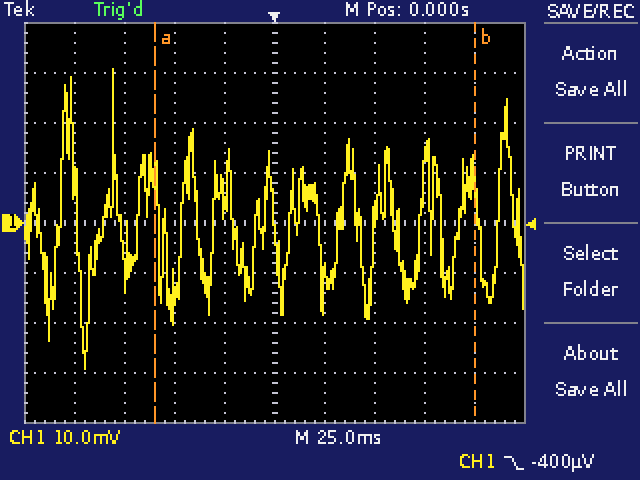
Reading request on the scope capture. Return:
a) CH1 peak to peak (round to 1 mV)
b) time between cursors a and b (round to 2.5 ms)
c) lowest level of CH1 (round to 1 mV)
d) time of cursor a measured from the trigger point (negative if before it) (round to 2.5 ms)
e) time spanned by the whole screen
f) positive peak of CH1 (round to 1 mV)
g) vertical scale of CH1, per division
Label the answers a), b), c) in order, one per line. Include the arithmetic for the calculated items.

a) 31 mV − (-29 mV) = 60 mV
b) 160.0 ms
c) -29 mV
d) -60.0 ms
e) 250 ms
f) 31 mV
g) 10 mV
